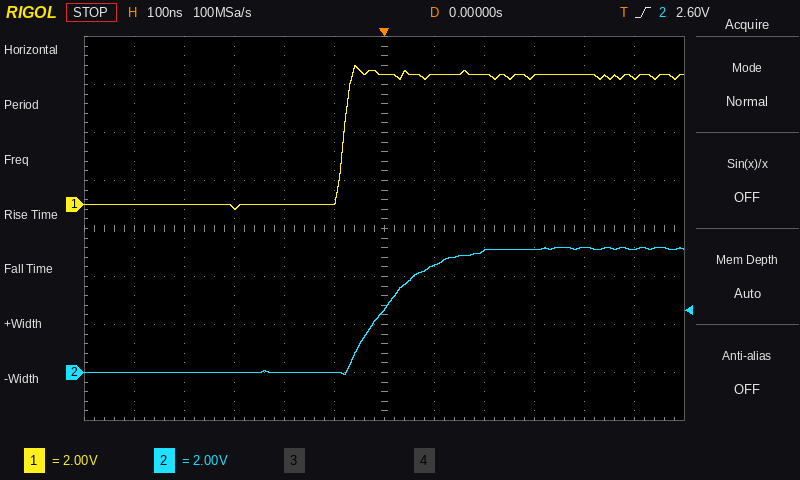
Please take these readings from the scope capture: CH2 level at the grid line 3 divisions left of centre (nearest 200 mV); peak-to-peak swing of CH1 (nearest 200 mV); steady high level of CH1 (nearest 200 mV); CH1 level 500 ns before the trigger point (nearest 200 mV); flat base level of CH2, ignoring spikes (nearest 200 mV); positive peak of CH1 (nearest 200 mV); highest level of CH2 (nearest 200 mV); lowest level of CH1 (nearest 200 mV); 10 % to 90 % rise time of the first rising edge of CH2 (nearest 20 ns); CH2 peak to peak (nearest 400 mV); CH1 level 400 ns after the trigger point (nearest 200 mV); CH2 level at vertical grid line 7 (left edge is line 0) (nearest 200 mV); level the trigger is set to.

0.0 V
6.0 V
5.4 V
0.0 V
0.0 V
5.8 V
5.2 V
-200 mV
180 ns
5.2 V
5.4 V
4.4 V
2.60 V
